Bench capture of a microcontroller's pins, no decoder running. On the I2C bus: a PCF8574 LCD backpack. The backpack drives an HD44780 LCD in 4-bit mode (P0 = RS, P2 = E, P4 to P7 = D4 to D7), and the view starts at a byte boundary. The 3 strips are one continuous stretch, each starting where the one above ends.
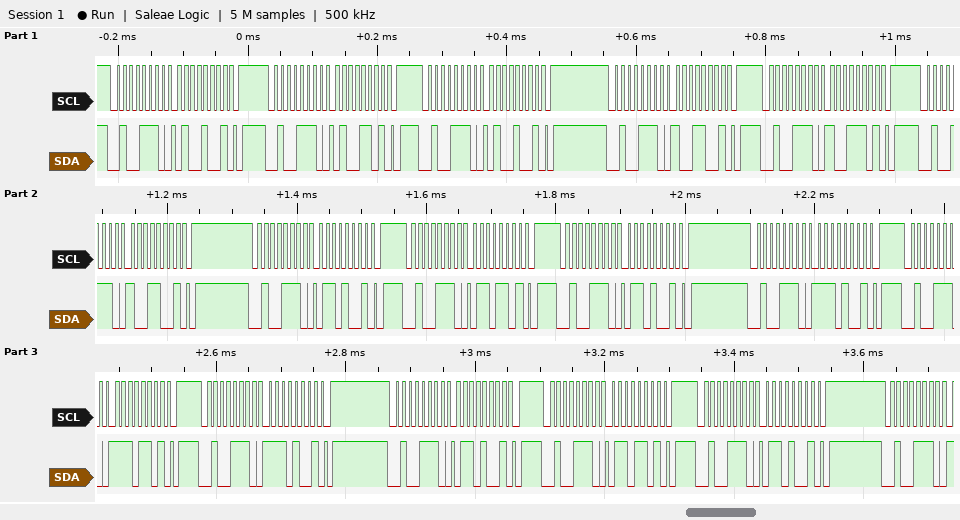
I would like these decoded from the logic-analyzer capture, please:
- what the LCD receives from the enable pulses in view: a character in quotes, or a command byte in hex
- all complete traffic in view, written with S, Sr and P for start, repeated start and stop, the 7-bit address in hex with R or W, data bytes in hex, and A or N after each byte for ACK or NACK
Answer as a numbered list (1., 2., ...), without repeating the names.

1. 'I' 'n'
2. S 27W A 49 A P S 27W A 4D A P S 27W A 49 A P S 27W A 99 A P S 27W A 9D A P S 27W A 99 A P S 27W A 69 A P S 27W A 6D A P S 27W A 69 A P S 27W A E9 A P S 27W A ED A P S 27W A E9 A P S 27W A 69 A P S 27W A 6D A P S 27W A 69 A P S 27W A
